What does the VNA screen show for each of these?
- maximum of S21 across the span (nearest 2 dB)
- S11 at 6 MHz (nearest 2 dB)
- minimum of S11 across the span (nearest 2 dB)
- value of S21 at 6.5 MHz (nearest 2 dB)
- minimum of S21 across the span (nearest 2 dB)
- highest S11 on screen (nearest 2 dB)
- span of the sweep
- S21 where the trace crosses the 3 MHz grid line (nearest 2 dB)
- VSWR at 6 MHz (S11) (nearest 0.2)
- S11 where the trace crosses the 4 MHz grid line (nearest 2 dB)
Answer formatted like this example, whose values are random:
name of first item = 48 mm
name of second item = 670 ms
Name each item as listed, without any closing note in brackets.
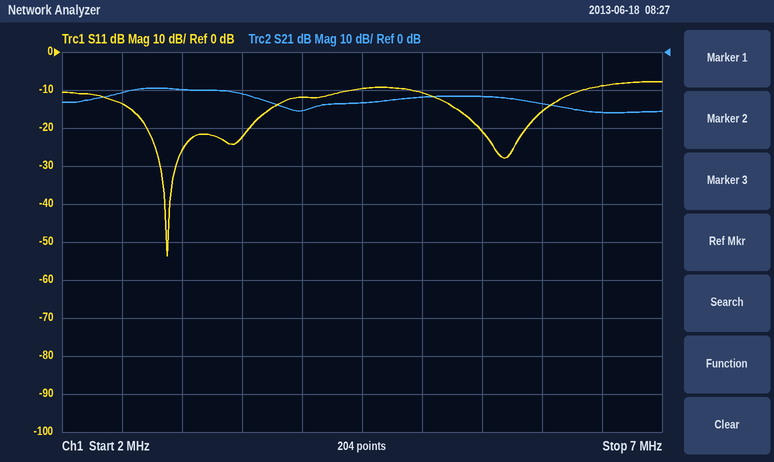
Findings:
maximum of S21 across the span = -10 dB
S11 at 6 MHz = -16 dB
minimum of S11 across the span = -54 dB
value of S21 at 6.5 MHz = -16 dB
minimum of S21 across the span = -16 dB
highest S11 on screen = -8 dB
span of the sweep = 5 MHz
S21 where the trace crosses the 3 MHz grid line = -10 dB
VSWR at 6 MHz (S11) = 1.4
S11 where the trace crosses the 4 MHz grid line = -12 dB
